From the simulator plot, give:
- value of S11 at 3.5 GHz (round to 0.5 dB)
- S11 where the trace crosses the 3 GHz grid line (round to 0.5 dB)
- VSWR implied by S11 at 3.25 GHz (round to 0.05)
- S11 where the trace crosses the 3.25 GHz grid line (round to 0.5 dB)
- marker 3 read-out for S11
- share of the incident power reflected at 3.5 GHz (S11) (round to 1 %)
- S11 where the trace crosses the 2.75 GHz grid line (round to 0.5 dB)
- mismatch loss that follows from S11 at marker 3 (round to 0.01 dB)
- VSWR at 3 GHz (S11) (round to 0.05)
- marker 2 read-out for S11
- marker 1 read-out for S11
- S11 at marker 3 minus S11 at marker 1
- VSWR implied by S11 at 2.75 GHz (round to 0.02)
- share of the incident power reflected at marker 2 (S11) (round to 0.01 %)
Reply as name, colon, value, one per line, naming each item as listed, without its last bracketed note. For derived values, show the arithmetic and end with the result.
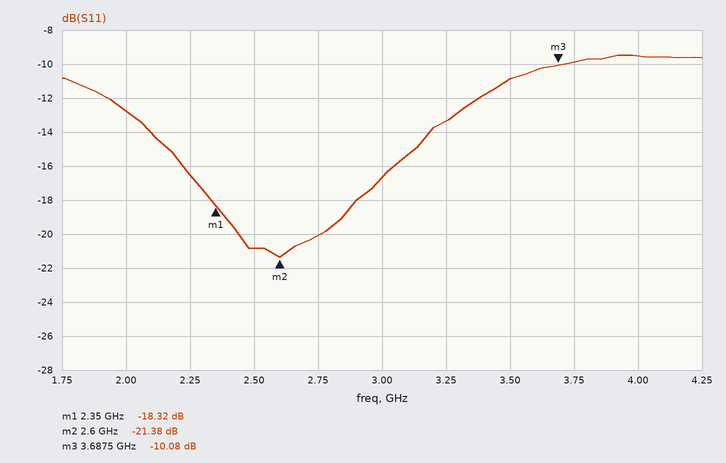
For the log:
value of S11 at 3.5 GHz: -11.0 dB
S11 where the trace crosses the 3 GHz grid line: -16.5 dB
VSWR implied by S11 at 3.25 GHz: |Γ| = 10^(-13.5/20) = 0.2113; VSWR = (1 + 0.2113)/(1 − 0.2113) ≈ 1.54, so 1.55 to the nearest 0.05
S11 where the trace crosses the 3.25 GHz grid line: -13.5 dB
marker 3 read-out for S11: -10.08 dB
share of the incident power reflected at 3.5 GHz (S11): 10^(-11/10) ≈ 8 %
S11 where the trace crosses the 2.75 GHz grid line: -20.0 dB
mismatch loss that follows from S11 at marker 3: −10 log10(1 − 10^(-10.08/10)) ≈ 0.45 dB
VSWR at 3 GHz (S11): |Γ| = 10^(-16.5/20) = 0.1496; VSWR = (1 + 0.1496)/(1 − 0.1496) ≈ 1.35
marker 2 read-out for S11: -21.38 dB
marker 1 read-out for S11: -18.32 dB
S11 at marker 3 minus S11 at marker 1: -10.08 − (-18.32) = 8.24 dB
VSWR implied by S11 at 2.75 GHz: |Γ| = 10^(-20/20) = 0.1000; VSWR = (1 + 0.1000)/(1 − 0.1000) ≈ 1.22
share of the incident power reflected at marker 2 (S11): 10^(-21.38/10) ≈ 0.73 %
